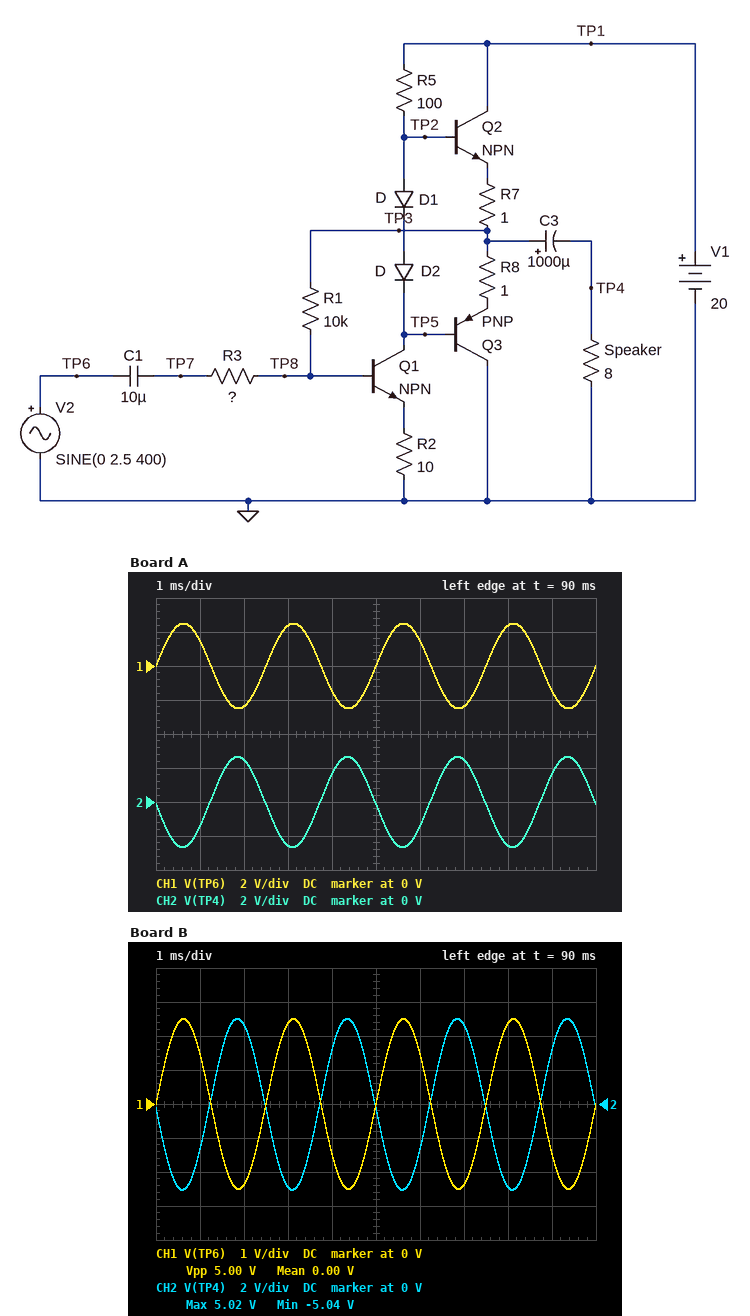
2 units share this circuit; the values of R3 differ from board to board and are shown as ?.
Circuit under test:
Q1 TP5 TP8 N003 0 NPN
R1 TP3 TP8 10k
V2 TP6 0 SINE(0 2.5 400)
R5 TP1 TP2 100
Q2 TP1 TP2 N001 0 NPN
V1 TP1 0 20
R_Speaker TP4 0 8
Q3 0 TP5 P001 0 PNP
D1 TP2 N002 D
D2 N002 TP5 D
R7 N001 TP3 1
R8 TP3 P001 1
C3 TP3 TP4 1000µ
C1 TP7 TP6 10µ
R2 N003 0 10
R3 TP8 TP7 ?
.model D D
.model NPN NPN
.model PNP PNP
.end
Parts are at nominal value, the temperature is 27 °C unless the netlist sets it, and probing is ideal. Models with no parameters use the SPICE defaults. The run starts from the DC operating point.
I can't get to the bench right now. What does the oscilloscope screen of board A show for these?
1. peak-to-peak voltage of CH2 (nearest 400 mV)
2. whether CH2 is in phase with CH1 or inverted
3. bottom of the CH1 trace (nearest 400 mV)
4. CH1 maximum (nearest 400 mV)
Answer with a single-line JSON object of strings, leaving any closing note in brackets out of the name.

{"peak-to-peak voltage of CH2": "5.2 V", "whether CH2 is in phase with CH1 or inverted": "inverted", "bottom of the CH1 trace": "-2.4 V", "CH1 maximum": "2.4 V"}
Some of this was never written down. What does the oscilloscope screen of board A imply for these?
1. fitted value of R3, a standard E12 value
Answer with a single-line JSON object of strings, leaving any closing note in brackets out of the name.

{"fitted value of R3, a standard E12 value": "3.3 kΩ"}
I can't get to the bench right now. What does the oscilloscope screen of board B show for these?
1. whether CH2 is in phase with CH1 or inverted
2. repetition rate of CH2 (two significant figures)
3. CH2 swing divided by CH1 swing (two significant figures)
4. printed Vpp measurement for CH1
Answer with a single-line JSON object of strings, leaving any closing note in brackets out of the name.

{"whether CH2 is in phase with CH1 or inverted": "inverted", "repetition rate of CH2": "400 Hz", "CH2 swing divided by CH1 swing": "2.0", "printed Vpp measurement for CH1": "5.00 V"}
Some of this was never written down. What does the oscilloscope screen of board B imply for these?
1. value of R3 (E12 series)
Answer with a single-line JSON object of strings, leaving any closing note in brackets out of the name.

{"value of R3": "1.5 kΩ"}
